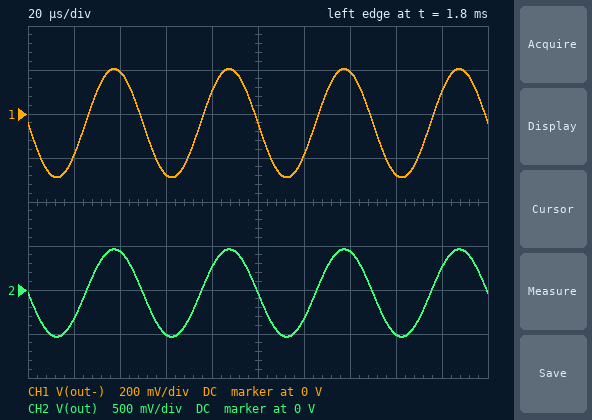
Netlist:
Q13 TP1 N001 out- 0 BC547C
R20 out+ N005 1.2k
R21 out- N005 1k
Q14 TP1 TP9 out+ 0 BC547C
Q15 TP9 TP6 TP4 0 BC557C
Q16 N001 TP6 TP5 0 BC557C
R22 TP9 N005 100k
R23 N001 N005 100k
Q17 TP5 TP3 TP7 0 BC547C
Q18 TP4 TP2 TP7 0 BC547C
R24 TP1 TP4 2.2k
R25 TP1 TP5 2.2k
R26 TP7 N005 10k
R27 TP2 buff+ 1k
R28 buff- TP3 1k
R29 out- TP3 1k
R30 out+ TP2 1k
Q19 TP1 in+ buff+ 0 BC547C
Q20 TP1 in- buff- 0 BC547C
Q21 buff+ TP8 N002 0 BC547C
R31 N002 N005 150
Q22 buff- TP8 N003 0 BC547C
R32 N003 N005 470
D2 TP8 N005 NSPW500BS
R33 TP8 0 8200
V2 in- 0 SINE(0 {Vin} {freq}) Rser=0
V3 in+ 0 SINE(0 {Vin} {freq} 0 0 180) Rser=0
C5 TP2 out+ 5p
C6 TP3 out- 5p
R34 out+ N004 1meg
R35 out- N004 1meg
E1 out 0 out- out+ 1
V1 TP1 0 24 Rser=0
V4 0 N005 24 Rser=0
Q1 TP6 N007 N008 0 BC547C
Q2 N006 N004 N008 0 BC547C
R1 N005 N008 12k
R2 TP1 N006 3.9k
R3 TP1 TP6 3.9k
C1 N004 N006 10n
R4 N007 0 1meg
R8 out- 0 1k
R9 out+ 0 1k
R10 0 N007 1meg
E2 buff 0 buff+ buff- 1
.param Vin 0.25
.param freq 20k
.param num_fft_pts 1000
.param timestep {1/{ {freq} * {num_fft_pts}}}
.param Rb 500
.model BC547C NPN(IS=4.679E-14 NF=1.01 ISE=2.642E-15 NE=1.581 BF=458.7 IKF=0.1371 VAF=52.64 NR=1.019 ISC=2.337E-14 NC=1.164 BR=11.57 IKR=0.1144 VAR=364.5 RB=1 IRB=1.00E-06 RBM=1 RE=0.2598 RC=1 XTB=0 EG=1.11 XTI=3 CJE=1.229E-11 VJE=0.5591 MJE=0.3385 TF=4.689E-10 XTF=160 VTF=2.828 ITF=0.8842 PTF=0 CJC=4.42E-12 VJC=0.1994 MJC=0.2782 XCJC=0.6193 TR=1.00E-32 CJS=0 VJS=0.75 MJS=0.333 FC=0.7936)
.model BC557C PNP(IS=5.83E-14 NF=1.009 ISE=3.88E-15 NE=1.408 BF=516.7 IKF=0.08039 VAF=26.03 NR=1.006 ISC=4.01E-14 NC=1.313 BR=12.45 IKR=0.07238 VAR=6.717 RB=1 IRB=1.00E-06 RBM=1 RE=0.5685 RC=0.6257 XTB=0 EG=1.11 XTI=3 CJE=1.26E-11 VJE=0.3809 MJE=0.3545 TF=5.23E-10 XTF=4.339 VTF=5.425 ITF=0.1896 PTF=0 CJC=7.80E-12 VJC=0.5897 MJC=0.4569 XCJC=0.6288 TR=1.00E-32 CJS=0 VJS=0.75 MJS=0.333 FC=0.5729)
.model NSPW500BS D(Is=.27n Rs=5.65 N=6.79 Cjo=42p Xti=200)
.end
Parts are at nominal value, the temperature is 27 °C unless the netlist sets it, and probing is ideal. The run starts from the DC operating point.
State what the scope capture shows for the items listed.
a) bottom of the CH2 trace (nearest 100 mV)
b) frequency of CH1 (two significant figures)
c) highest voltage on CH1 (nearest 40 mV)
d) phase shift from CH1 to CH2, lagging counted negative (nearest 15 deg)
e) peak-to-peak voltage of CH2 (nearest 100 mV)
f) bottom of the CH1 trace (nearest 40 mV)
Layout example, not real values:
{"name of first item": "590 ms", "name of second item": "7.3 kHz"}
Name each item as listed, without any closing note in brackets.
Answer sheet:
{"bottom of the CH2 trace": "-500 mV", "frequency of CH1": "20 kHz", "highest voltage on CH1": "200 mV", "phase shift from CH1 to CH2, lagging counted negative": "0 deg", "peak-to-peak voltage of CH2": "1.0 V", "bottom of the CH1 trace": "-280 mV"}
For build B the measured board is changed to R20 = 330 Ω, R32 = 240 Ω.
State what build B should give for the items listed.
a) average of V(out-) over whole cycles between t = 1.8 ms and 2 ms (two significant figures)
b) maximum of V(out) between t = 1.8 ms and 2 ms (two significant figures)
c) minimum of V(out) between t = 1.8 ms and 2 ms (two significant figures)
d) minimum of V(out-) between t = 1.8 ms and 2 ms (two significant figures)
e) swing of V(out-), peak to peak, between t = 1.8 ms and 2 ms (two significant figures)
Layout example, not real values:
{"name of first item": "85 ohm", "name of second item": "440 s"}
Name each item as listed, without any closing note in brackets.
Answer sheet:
{"average of V(out-) over whole cycles between t = 1.8 ms and 2 ms": "-88 mV", "maximum of V(out) between t = 1.8 ms and 2 ms": "490 mV", "minimum of V(out) between t = 1.8 ms and 2 ms": "-510 mV", "minimum of V(out-) between t = 1.8 ms and 2 ms": "-360 mV", "swing of V(out-), peak to peak, between t = 1.8 ms and 2 ms": "550 mV"}
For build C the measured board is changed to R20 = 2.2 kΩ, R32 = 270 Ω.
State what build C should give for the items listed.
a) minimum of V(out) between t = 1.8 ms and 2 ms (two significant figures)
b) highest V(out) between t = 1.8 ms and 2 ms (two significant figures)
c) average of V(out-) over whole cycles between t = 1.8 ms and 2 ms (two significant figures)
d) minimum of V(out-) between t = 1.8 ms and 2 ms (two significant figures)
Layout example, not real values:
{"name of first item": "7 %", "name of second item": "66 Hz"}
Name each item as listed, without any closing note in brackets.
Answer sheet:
{"minimum of V(out) between t = 1.8 ms and 2 ms": "-520 mV", "highest V(out) between t = 1.8 ms and 2 ms": "480 mV", "average of V(out-) over whole cycles between t = 1.8 ms and 2 ms": "-26 mV", "minimum of V(out-) between t = 1.8 ms and 2 ms": "-270 mV"}
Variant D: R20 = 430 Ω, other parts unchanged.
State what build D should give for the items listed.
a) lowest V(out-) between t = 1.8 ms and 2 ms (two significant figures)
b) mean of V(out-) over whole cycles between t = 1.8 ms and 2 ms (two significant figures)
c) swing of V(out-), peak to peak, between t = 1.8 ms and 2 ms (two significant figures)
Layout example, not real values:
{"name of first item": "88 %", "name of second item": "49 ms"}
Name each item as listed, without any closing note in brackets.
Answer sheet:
{"lowest V(out-) between t = 1.8 ms and 2 ms": "-340 mV", "mean of V(out-) over whole cycles between t = 1.8 ms and 2 ms": "-78 mV", "swing of V(out-), peak to peak, between t = 1.8 ms and 2 ms": "530 mV"}
